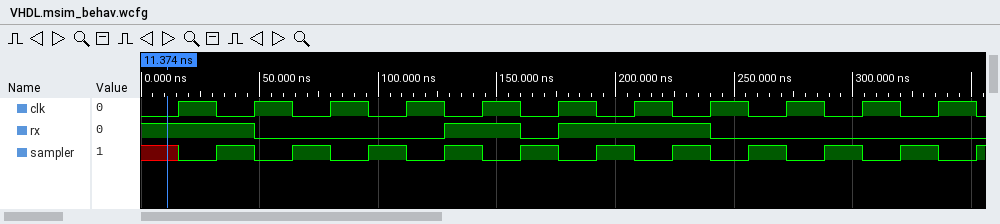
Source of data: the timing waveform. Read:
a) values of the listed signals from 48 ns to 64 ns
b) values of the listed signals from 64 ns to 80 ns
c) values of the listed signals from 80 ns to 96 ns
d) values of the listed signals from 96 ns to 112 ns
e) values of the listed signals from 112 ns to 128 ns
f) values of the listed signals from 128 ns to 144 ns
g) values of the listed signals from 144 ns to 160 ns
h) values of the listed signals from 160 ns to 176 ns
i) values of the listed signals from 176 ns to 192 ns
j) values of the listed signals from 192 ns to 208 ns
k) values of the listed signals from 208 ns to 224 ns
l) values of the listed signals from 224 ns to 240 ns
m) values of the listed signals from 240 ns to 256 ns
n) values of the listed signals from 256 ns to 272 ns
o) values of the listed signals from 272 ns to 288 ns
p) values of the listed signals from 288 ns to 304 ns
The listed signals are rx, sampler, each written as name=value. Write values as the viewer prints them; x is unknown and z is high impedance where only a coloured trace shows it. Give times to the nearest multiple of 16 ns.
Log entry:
rx=0, sampler=0
rx=0, sampler=1
rx=0, sampler=0
rx=0, sampler=1
rx=0, sampler=0
rx=1, sampler=1
rx=1, sampler=0
rx=0, sampler=1
rx=1, sampler=0
rx=1, sampler=1
rx=1, sampler=0
rx=1, sampler=1
rx=0, sampler=0
rx=0, sampler=1
rx=0, sampler=0
rx=0, sampler=1
